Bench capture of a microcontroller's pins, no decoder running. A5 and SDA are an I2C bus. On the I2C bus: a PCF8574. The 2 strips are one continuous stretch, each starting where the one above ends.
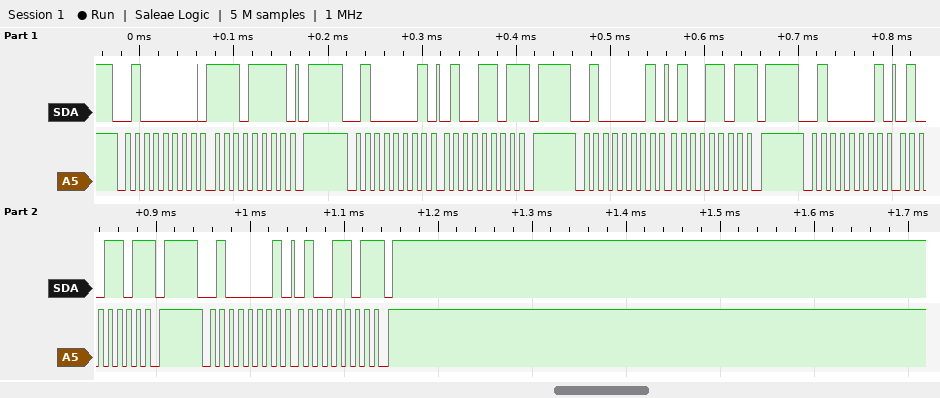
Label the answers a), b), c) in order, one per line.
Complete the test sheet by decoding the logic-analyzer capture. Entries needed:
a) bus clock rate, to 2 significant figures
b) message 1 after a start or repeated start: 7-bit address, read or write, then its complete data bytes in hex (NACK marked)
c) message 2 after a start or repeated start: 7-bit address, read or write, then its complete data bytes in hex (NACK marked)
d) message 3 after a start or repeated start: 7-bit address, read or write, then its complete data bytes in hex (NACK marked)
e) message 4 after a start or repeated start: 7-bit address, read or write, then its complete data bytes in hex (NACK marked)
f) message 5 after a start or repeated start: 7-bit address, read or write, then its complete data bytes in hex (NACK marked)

a) 100 kHz
b) 0x20 write: EF
c) 0x20 read: 4D NACK
d) 0x20 read: 4D NACK
e) 0x20 read: 4D NACK
f) 0x20 read: 4D NACK
